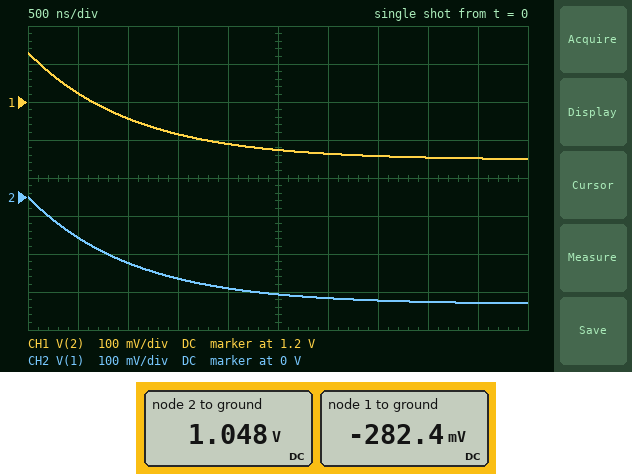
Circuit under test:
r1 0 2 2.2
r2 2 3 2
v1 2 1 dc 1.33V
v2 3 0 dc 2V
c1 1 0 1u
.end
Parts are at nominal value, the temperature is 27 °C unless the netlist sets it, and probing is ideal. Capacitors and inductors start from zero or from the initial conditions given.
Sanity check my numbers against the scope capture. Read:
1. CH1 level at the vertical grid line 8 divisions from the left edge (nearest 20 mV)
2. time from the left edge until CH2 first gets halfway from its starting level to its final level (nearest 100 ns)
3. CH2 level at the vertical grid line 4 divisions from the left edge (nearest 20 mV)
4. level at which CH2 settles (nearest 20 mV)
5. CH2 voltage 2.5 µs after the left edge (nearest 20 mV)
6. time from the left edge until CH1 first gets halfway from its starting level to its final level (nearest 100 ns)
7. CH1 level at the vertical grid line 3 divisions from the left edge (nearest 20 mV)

1.06 V
700 ns
-240 mV
-280 mV
-260 mV
700 ns
1.12 V
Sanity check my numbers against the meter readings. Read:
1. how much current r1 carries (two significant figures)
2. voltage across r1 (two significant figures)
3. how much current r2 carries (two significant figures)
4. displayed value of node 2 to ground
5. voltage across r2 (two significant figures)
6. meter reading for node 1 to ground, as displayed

480 mA
1.0 V
480 mA
1.048 V
950 mV
-282.4 mV
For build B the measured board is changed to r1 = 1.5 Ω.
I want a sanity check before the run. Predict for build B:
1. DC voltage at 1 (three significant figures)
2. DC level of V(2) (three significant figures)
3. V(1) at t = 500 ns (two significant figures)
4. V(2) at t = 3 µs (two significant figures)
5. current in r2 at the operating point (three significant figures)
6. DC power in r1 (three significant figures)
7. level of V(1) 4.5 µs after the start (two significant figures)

-473 mV
857 mV
-210 mV
870 mV
571 mA
490 mW
-470 mV
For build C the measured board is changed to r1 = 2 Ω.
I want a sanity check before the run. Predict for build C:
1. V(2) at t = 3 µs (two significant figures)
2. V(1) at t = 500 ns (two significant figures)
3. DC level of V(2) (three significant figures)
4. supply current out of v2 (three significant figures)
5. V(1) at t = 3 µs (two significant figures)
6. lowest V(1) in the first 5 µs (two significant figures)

1.0 V
-130 mV
1.00 V
500 mA
-310 mV
-330 mV
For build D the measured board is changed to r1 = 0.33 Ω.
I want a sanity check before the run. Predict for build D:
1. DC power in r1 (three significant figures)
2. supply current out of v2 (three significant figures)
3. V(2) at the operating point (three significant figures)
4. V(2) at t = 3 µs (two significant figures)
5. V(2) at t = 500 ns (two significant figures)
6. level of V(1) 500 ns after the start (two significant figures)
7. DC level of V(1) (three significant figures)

243 mW
858 mA
283 mV
280 mV
460 mV
-870 mV
-1.05 V
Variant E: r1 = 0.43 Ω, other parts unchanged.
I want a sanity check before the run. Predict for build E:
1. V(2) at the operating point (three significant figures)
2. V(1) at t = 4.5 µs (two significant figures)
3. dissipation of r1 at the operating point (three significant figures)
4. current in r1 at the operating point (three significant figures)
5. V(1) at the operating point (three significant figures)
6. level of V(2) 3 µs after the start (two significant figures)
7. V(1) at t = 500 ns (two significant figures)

354 mV
-980 mV
291 mW
823 mA
-976 mV
350 mV
-740 mV
